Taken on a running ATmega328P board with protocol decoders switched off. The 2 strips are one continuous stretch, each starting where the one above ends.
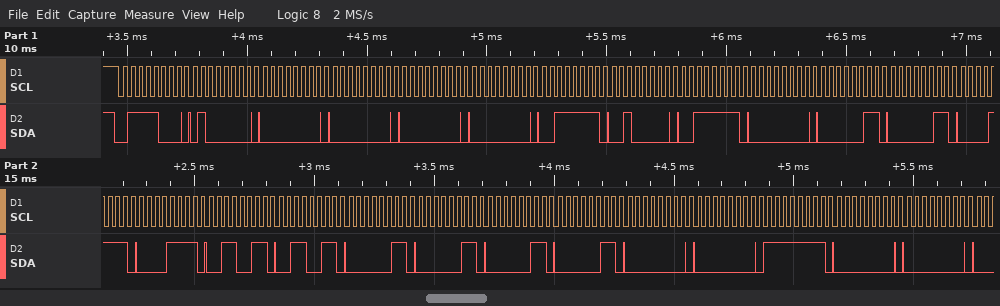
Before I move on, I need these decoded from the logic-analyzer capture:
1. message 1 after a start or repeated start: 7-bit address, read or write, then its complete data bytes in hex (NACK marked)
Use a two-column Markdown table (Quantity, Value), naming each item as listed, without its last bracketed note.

| Quantity | Value |
|---|---|
| message 1 after a start or repeated start: 7-bit address, read or write, then its complete data bytes in hex | 0x3C write: 40 00 00 00 00 3F 20 3F 00 03 03 0F 0F 33 33 03 03 03 03 00 00 FF 00 00 |
